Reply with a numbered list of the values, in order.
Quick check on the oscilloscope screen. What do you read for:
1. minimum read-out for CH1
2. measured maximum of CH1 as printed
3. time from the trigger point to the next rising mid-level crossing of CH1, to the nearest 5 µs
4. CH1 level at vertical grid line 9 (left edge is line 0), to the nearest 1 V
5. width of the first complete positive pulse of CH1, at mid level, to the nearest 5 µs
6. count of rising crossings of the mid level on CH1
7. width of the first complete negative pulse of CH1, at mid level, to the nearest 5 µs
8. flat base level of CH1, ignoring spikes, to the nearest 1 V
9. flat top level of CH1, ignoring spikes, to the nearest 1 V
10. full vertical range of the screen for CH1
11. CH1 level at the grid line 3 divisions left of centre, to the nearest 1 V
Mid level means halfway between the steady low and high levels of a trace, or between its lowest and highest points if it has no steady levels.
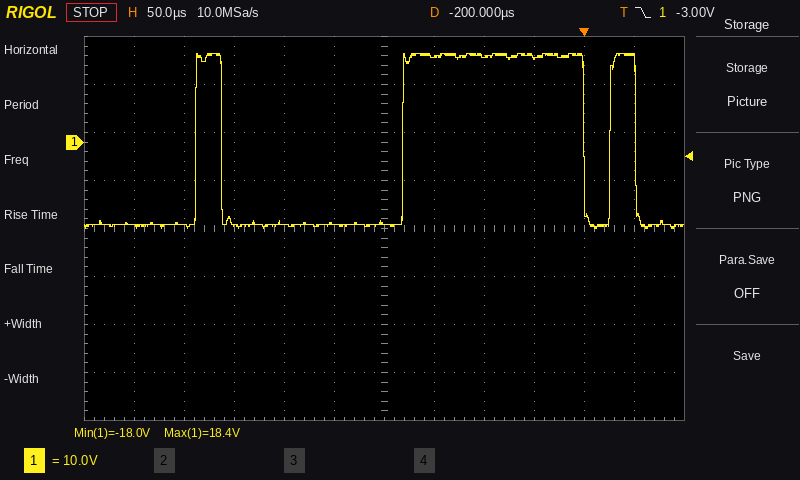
1. -18.0 V
2. 18.4 V
3. 25 µs
4. 18 V
5. 25 µs
6. 3
7. 180 µs
8. -17 V
9. 18 V
10. 80 V
11. -17 V
